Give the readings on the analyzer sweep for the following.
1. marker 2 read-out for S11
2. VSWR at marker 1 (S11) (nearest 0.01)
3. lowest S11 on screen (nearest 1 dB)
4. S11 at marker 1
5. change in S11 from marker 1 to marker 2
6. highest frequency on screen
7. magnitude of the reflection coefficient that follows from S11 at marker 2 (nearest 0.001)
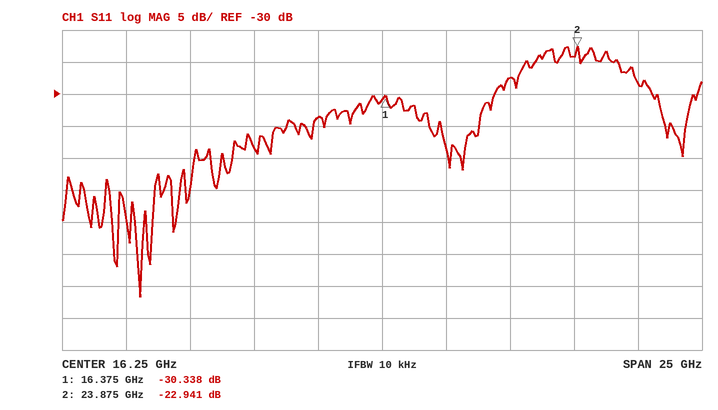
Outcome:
-22.941 dB
1.06
-62 dB
-30.338 dB
7.397 dB
28.75 GHz
0.071
